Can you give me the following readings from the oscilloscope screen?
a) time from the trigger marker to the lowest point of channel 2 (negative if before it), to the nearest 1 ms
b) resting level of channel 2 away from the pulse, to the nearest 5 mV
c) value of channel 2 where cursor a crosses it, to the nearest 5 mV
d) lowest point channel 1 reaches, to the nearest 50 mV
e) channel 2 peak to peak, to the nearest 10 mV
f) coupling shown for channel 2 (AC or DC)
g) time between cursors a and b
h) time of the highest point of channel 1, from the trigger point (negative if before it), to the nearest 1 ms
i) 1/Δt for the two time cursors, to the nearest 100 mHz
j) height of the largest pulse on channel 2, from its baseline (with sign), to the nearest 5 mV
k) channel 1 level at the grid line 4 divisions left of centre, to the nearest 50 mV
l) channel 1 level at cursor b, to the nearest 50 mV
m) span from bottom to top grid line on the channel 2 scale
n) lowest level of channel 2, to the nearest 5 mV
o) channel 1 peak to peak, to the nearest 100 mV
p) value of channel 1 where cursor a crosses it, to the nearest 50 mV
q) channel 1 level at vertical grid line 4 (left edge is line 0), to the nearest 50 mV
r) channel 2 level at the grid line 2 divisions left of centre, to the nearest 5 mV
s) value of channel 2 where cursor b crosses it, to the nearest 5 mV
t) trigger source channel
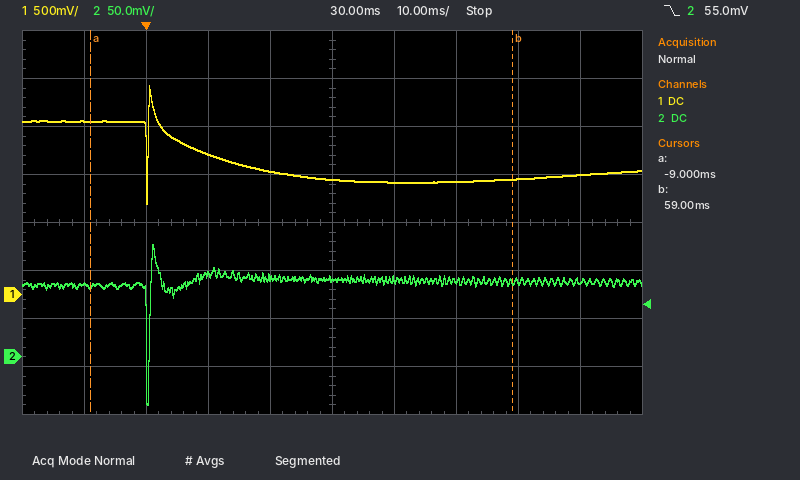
0 ms
80 mV
75 mV
950 mV
170 mV
DC
68 ms
+1 ms
14.7 Hz
-130 mV
1.80 V
1.20 V
400 mV
-50 mV
1.20 V
1.80 V
1.30 V
85 mV
80 mV
channel 2
